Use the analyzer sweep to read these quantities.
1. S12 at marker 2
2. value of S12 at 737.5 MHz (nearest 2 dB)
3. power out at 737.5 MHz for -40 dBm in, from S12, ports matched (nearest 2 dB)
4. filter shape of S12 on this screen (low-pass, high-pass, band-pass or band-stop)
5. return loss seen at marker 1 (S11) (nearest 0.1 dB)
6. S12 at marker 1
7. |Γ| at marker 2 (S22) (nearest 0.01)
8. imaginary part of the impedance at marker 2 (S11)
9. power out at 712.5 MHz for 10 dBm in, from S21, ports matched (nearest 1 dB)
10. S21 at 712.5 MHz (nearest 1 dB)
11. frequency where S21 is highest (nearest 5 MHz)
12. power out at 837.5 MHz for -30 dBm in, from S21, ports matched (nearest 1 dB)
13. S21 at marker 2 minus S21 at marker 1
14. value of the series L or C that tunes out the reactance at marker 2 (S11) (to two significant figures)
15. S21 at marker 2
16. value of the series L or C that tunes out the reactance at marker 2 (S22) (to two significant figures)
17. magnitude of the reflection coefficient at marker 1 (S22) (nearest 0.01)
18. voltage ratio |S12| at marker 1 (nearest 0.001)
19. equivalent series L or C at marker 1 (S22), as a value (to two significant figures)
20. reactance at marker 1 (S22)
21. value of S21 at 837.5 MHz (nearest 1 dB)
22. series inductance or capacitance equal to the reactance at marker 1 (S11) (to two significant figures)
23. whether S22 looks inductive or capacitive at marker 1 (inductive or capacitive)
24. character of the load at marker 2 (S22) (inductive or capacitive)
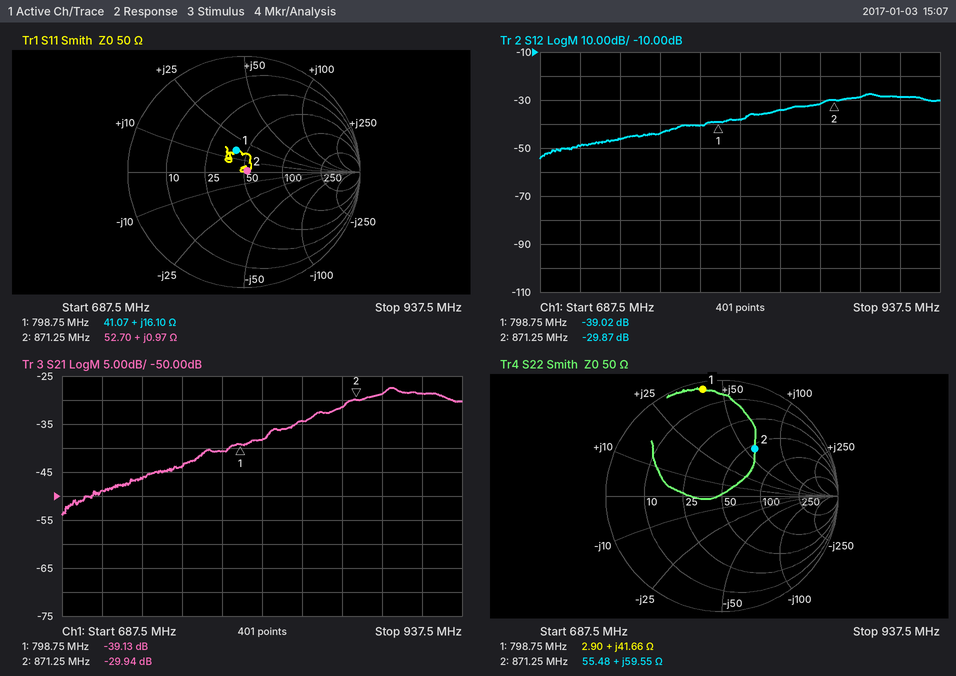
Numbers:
-29.87 dB
-46 dB
-86 dBm
high-pass
14.0 dB
-39.02 dB
0.49
+0.97 Ω
-39 dBm
-49 dB
895 MHz
-64 dBm
9.19 dB
190 pF
-29.94 dB
3.1 pF
0.93
0.011
8.3 nH
+41.66 Ω
-34 dB
3.2 nH
inductive
inductive
